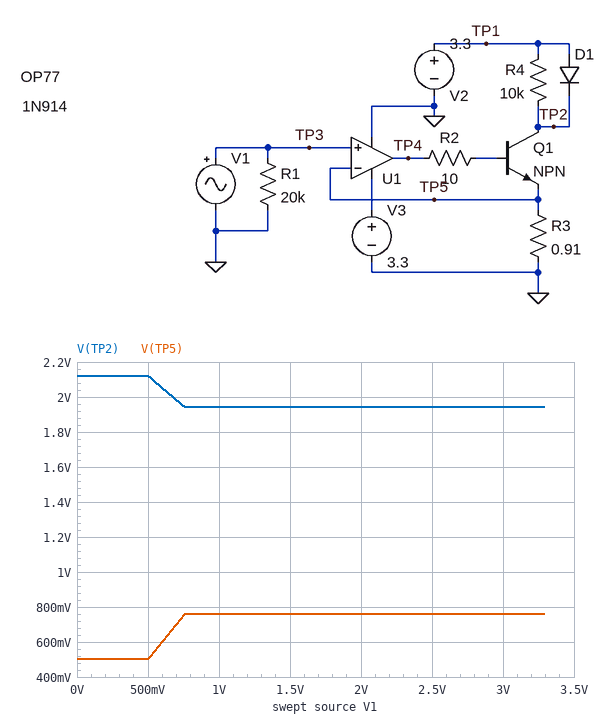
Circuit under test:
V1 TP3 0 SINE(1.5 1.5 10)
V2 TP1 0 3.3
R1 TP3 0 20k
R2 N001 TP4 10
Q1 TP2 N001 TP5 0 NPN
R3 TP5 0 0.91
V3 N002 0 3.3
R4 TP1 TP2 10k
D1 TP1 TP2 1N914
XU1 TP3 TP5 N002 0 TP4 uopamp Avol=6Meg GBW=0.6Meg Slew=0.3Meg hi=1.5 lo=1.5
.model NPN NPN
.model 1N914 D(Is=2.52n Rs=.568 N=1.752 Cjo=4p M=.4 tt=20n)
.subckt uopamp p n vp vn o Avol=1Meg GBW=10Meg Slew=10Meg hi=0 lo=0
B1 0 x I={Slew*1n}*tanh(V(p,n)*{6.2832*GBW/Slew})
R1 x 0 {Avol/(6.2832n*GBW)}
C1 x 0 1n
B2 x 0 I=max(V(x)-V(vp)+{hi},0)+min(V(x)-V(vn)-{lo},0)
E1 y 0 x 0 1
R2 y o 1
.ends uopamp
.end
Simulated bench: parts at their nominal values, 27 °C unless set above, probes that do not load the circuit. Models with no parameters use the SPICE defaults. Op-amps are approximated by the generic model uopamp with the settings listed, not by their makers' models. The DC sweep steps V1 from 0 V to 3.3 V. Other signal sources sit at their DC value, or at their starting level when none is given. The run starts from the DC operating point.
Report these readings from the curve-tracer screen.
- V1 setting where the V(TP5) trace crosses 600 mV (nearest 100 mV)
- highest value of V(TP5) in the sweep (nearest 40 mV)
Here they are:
600 mV
760 mV
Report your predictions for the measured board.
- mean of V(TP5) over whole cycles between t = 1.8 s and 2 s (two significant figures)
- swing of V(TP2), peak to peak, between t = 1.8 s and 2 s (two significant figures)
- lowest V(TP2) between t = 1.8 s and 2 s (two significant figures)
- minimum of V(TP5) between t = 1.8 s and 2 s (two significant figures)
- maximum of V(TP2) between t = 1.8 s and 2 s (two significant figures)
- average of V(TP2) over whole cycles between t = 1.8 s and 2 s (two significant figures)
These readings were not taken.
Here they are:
680 mV
180 mV
1.9 V
500 mV
2.1 V
2.0 V
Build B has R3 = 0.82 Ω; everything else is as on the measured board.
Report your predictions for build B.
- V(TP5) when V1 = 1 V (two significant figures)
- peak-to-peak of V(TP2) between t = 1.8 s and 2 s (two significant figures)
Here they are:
750 mV
190 mV
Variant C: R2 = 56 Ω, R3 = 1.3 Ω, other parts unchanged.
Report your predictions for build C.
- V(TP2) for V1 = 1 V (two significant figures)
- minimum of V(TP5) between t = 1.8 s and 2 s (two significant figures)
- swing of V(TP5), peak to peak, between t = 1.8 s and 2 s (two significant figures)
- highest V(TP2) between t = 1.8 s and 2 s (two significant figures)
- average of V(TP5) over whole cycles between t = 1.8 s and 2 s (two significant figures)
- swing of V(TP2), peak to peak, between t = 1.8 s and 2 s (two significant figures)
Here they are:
2.2 V
400 mV
200 mV
2.3 V
550 mV
110 mV
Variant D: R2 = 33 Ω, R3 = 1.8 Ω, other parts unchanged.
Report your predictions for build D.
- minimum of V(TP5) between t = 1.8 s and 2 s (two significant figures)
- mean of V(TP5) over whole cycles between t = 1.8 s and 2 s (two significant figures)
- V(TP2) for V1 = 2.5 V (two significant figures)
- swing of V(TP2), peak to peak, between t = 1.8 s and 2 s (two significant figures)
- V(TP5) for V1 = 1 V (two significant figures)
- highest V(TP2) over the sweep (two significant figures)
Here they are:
490 mV
660 mV
2.2 V
95 mV
730 mV
2.3 V
